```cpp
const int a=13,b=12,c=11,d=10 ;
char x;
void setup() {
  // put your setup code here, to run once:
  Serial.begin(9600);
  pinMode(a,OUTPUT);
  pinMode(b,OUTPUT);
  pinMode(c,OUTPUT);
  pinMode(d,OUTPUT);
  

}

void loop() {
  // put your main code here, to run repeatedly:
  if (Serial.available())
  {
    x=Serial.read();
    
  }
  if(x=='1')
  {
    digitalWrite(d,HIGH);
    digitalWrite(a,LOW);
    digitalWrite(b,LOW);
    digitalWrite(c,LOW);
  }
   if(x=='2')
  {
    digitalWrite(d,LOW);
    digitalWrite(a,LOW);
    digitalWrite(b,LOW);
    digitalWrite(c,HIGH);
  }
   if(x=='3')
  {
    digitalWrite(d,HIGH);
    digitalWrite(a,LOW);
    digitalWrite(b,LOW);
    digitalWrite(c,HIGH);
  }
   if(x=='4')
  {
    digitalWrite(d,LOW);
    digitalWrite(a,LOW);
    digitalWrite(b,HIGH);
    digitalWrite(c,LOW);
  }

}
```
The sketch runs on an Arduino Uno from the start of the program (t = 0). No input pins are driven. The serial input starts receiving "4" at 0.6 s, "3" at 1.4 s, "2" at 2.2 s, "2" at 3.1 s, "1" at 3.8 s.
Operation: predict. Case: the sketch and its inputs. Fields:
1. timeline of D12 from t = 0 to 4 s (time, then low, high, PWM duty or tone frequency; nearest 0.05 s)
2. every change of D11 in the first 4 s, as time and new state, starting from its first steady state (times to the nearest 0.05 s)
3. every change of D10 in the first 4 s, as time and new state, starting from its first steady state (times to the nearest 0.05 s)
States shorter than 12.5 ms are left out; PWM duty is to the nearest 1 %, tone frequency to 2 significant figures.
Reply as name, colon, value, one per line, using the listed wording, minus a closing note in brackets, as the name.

timeline of D12 from t = 0 to 4 s: 0 s low; 0.6 s high; 1.4 s low
every change of D11 in the first 4 s, as time and new state, starting from its first steady state: 0 s low; 1.4 s high; 3.8 s low
every change of D10 in the first 4 s, as time and new state, starting from its first steady state: 0 s low; 1.4 s high; 2.2 s low; 3.8 s high
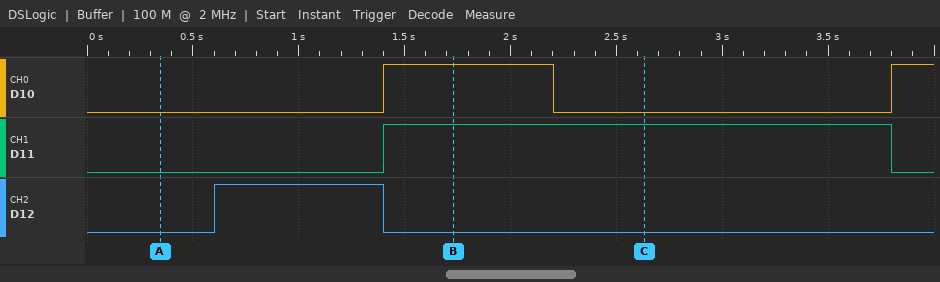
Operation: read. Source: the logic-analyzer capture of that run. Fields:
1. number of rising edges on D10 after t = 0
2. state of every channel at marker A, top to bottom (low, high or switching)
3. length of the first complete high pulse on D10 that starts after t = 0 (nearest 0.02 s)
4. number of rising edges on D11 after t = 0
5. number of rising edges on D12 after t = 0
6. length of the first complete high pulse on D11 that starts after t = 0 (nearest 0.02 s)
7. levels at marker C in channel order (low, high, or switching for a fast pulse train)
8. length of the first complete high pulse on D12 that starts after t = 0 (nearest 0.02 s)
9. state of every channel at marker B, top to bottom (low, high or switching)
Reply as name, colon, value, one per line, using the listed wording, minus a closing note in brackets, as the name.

number of rising edges on D10 after t = 0: 2
state of every channel at marker A, top to bottom: D10 low, D11 low, D12 low
length of the first complete high pulse on D10 that starts after t = 0: 0.80 s
number of rising edges on D11 after t = 0: 1
number of rising edges on D12 after t = 0: 1
length of the first complete high pulse on D11 that starts after t = 0: 2.40 s
levels at marker C in channel order: D10 low, D11 high, D12 low
length of the first complete high pulse on D12 that starts after t = 0: 0.80 s
state of every channel at marker B, top to bottom: D10 high, D11 high, D12 low
